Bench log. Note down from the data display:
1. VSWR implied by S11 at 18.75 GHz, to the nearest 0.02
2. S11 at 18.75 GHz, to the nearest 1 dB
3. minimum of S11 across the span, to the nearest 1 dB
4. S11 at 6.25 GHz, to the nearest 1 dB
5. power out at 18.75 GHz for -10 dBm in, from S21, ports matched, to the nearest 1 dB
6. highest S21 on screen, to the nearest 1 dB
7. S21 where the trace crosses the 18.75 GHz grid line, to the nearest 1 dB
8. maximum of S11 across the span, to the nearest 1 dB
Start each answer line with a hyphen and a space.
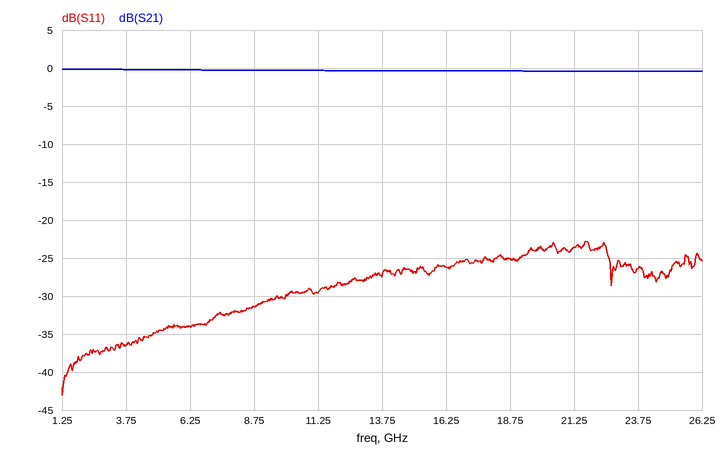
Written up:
- 1.12
- -25 dB
- -43 dB
- -34 dB
- -10 dBm
- 0 dB
- 0 dB
- -23 dB
